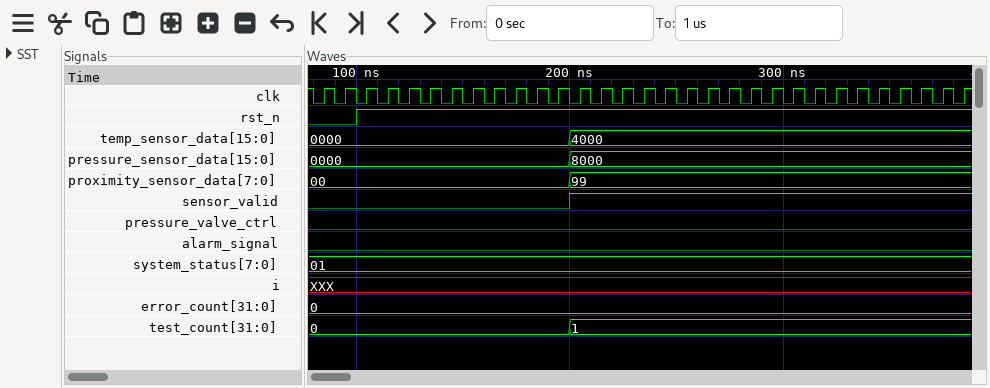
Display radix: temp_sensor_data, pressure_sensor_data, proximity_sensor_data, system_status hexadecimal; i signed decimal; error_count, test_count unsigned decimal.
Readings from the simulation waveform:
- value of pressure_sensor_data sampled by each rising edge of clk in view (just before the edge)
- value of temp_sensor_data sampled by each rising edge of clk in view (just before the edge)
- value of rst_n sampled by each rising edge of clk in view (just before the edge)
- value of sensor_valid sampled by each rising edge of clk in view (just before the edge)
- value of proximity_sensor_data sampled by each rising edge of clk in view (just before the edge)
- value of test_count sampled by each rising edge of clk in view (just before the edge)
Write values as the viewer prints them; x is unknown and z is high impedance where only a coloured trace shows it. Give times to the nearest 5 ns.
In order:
0000, 0000, 0000, 0000, 0000, 0000, 0000, 0000, 0000, 0000, 0000, 0000, 8000, 8000, 8000, 8000, 8000, 8000, 8000, 8000, 8000, 8000, 8000, 8000, 8000, 8000, 8000, 8000, 8000, 8000, 8000
0000, 0000, 0000, 0000, 0000, 0000, 0000, 0000, 0000, 0000, 0000, 0000, 4000, 4000, 4000, 4000, 4000, 4000, 4000, 4000, 4000, 4000, 4000, 4000, 4000, 4000, 4000, 4000, 4000, 4000, 4000
0 0 1 1 1 1 1 1 1 1 1 1 1 1 1 1 1 1 1 1 1 1 1 1 1 1 1 1 1 1 1
0 0 0 0 0 0 0 0 0 0 0 0 1 1 1 1 1 1 1 1 1 1 1 1 1 1 1 1 1 1 1
00, 00, 00, 00, 00, 00, 00, 00, 00, 00, 00, 00, 99, 99, 99, 99, 99, 99, 99, 99, 99, 99, 99, 99, 99, 99, 99, 99, 99, 99, 99
0, 0, 0, 0, 0, 0, 0, 0, 0, 0, 0, 0, 1, 1, 1, 1, 1, 1, 1, 1, 1, 1, 1, 1, 1, 1, 1, 1, 1, 1, 1
